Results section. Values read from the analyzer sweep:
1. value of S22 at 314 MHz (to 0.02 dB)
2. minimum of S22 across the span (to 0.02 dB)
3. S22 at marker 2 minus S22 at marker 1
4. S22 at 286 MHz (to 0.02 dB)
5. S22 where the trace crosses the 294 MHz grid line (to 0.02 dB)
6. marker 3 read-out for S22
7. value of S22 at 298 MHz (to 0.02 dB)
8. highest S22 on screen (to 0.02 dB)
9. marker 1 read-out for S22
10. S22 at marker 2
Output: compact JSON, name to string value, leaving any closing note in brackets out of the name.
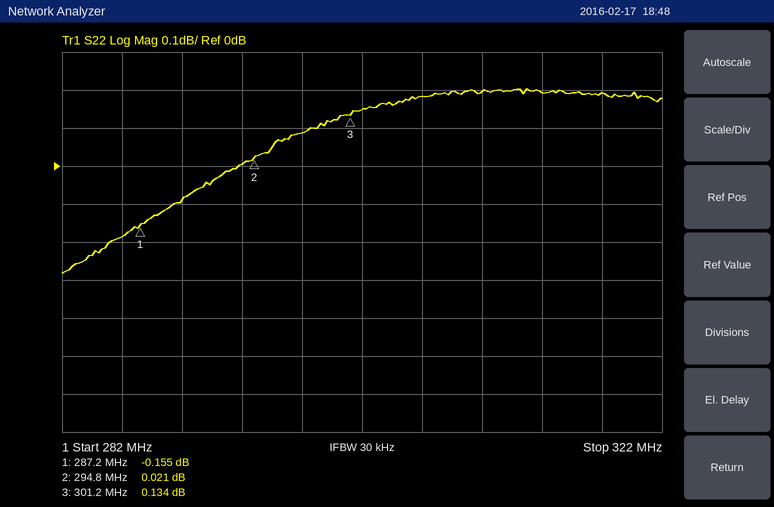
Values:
{"value of S22 at 314 MHz": "0.20 dB", "minimum of S22 across the span": "-0.28 dB", "S22 at marker 2 minus S22 at marker 1": "0.176 dB", "S22 at 286 MHz": "-0.18 dB", "S22 where the trace crosses the 294 MHz grid line": "0.00 dB", "marker 3 read-out for S22": "0.134 dB", "value of S22 at 298 MHz": "0.08 dB", "highest S22 on screen": "0.20 dB", "marker 1 read-out for S22": "-0.155 dB", "S22 at marker 2": "0.021 dB"}
